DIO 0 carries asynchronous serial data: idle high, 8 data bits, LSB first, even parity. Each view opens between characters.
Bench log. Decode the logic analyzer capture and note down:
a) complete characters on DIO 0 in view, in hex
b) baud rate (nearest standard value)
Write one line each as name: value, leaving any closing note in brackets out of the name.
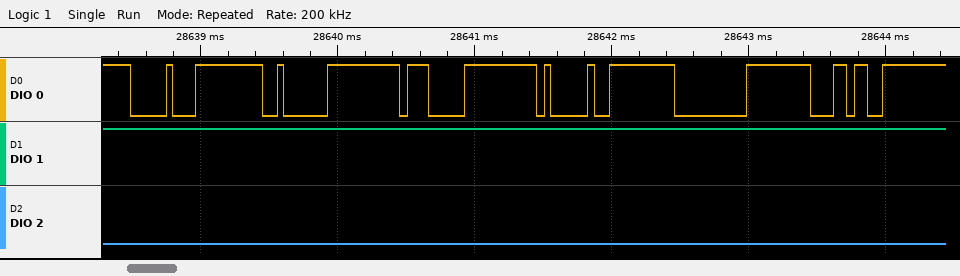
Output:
complete characters on DIO 0 in view, in hex: 10, 02, 07, 41, 00, 6C
baud rate: 19200 baud
